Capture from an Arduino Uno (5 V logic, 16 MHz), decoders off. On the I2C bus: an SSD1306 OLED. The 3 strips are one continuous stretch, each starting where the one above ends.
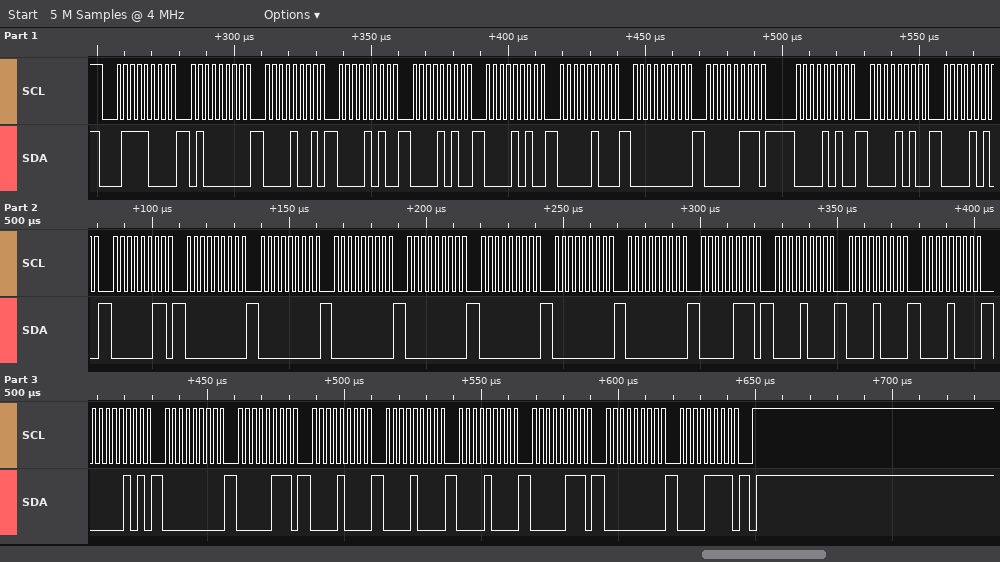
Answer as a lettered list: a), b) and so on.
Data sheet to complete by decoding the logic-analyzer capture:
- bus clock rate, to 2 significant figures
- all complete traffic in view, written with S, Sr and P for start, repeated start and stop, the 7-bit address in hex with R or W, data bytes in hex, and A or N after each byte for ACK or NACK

a) 400 kHz
b) S 3CW A 40 A 09 A 0A A 0A A 0A A 04 A 00 A 07 A 0A A 0A A 0A A 03 A 00 A 00 A 00 A 00 A 00 A 00 A 00 A 07 A 08 A 08 A 08 A 05 A 00 A 07 A 08 A 08 A 08 A 07 A 00 A 0F A P
